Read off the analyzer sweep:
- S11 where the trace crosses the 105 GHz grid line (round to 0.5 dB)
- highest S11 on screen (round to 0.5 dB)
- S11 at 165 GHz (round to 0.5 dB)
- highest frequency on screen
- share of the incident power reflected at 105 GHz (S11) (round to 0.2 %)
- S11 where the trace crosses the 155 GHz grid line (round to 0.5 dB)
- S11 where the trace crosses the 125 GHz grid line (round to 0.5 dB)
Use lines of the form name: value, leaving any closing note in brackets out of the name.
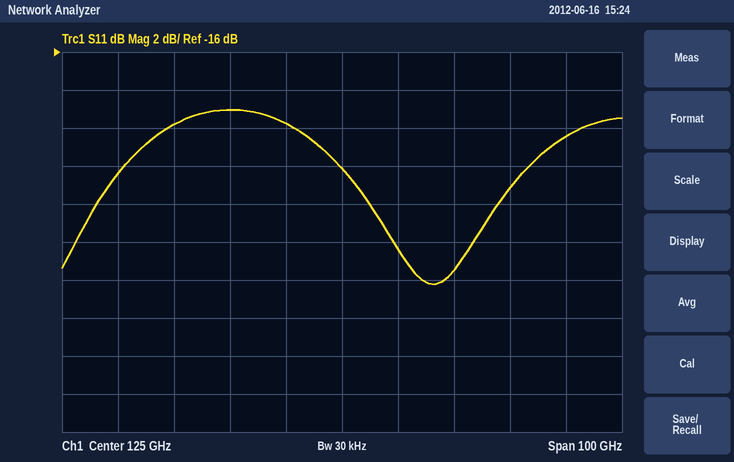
S11 where the trace crosses the 105 GHz grid line: -19.0 dB
highest S11 on screen: -19.0 dB
S11 at 165 GHz: -20.5 dB
highest frequency on screen: 175 GHz
share of the incident power reflected at 105 GHz (S11): 1.2 %
S11 where the trace crosses the 155 GHz grid line: -23.0 dB
S11 where the trace crosses the 125 GHz grid line: -22.0 dB
